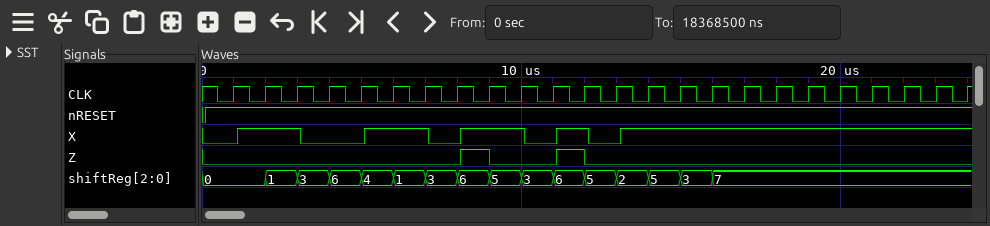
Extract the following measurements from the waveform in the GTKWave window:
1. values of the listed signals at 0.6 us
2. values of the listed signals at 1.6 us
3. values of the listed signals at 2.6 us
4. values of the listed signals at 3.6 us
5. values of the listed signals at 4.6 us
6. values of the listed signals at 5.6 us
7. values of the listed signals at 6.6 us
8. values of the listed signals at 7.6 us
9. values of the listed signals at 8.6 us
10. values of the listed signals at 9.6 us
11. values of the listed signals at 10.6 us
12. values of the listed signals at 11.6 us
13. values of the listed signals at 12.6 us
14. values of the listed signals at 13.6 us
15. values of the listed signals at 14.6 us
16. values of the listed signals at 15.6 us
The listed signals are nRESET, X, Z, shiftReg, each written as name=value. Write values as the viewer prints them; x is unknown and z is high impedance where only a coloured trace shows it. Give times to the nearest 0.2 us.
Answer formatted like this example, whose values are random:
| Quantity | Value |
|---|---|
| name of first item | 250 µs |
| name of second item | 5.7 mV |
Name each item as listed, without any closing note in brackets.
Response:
| Quantity | Value |
|---|---|
| values of the listed signals at 0.6 us | nRESET=1, X=0, Z=0, shiftReg=0 |
| values of the listed signals at 1.6 us | nRESET=1, X=1, Z=0, shiftReg=0 |
| values of the listed signals at 2.6 us | nRESET=1, X=1, Z=0, shiftReg=1 |
| values of the listed signals at 3.6 us | nRESET=1, X=0, Z=0, shiftReg=3 |
| values of the listed signals at 4.6 us | nRESET=1, X=0, Z=0, shiftReg=6 |
| values of the listed signals at 5.6 us | nRESET=1, X=1, Z=0, shiftReg=4 |
| values of the listed signals at 6.6 us | nRESET=1, X=1, Z=0, shiftReg=1 |
| values of the listed signals at 7.6 us | nRESET=1, X=0, Z=0, shiftReg=3 |
| values of the listed signals at 8.6 us | nRESET=1, X=1, Z=1, shiftReg=6 |
| values of the listed signals at 9.6 us | nRESET=1, X=1, Z=0, shiftReg=5 |
| values of the listed signals at 10.6 us | nRESET=1, X=0, Z=0, shiftReg=3 |
| values of the listed signals at 11.6 us | nRESET=1, X=1, Z=1, shiftReg=6 |
| values of the listed signals at 12.6 us | nRESET=1, X=0, Z=0, shiftReg=5 |
| values of the listed signals at 13.6 us | nRESET=1, X=1, Z=0, shiftReg=2 |
| values of the listed signals at 14.6 us | nRESET=1, X=1, Z=0, shiftReg=5 |
| values of the listed signals at 15.6 us | nRESET=1, X=1, Z=0, shiftReg=3 |
